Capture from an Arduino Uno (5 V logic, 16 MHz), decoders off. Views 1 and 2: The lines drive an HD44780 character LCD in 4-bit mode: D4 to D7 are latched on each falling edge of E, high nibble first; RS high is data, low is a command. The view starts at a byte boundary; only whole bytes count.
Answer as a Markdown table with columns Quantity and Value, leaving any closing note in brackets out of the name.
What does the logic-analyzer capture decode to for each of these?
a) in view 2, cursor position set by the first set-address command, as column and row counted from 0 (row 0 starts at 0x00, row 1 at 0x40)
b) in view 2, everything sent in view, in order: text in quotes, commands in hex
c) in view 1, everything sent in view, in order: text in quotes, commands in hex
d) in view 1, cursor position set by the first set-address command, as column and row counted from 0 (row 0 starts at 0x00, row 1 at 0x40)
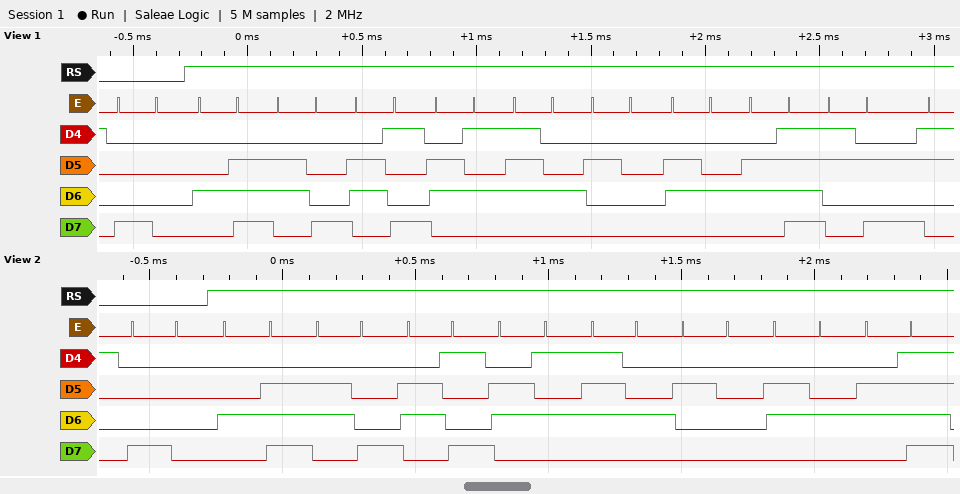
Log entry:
| Quantity | Value |
|---|---|
| in view 2, cursor position set by the first set-address command, as column and row counted from 0 | column 0, row 0 |
| in view 2, everything sent in view, in order: text in quotes, commands in hex | 0x80 "Nhiet do" |
| in view 1, everything sent in view, in order: text in quotes, commands in hex | 0x80 "Nhiet do:" |
| in view 1, cursor position set by the first set-address command, as column and row counted from 0 | column 0, row 0 |
